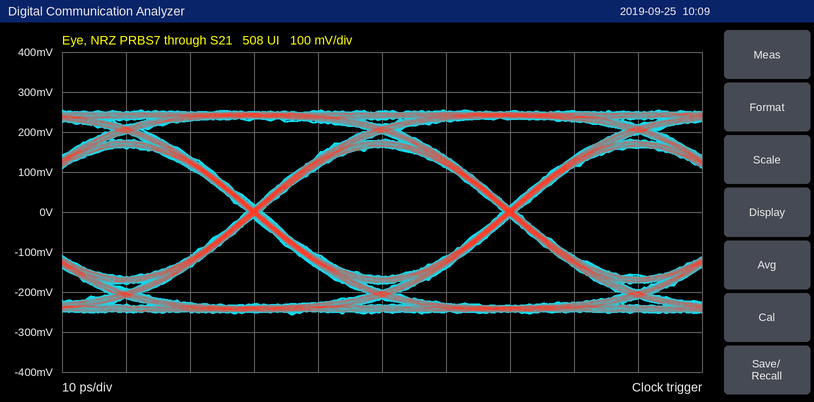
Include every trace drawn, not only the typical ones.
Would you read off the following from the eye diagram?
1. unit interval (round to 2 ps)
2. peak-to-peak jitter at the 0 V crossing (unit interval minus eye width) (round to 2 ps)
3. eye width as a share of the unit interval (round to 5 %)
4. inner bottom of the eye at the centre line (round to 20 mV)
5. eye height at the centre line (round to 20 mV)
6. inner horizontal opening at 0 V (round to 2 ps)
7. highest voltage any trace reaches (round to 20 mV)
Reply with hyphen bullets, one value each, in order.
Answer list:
- 40 ps
- 2 ps
- 95 %
- -160 mV
- 320 mV
- 38 ps
- 260 mV
